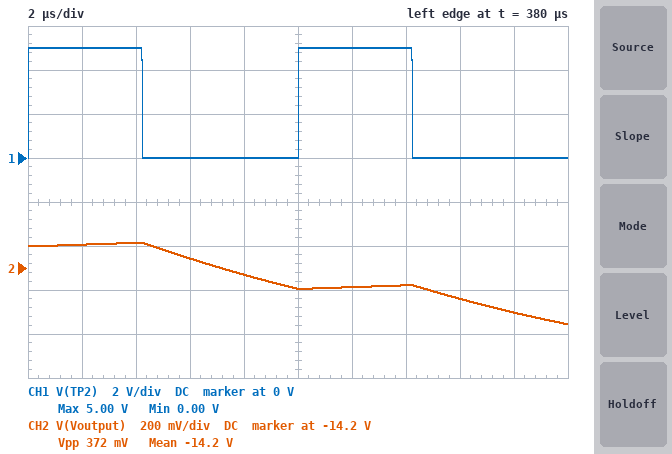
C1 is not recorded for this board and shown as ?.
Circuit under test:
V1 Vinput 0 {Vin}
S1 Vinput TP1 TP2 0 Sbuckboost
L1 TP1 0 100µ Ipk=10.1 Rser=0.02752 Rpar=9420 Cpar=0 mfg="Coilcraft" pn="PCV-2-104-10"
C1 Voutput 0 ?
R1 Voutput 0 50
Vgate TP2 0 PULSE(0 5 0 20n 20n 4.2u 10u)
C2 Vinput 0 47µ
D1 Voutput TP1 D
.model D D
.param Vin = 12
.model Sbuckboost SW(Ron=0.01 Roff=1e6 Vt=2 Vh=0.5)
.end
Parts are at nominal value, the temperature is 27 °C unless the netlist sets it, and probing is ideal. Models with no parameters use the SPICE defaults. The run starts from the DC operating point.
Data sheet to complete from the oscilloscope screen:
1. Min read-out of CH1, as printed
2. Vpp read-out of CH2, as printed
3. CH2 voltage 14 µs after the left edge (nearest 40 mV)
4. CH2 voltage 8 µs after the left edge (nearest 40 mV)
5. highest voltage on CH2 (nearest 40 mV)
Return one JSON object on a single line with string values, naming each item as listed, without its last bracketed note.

{"Min read-out of CH1, as printed": "0.00 V", "Vpp read-out of CH2, as printed": "372 mV", "CH2 voltage 14 µs after the left edge": "-14.28 V", "CH2 voltage 8 µs after the left edge": "-14.24 V", "highest voltage on CH2": "-14.08 V"}
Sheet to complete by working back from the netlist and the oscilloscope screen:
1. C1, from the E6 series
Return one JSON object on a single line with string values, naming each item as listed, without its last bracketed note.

{"C1, from the E6 series": "68 µF"}
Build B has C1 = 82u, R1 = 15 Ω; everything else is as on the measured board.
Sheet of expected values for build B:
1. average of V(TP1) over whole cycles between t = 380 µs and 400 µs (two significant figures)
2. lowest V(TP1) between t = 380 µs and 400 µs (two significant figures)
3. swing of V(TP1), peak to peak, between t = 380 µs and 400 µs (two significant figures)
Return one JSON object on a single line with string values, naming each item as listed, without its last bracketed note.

{"average of V(TP1) over whole cycles between t = 380 µs and 400 µs": "-2.7 V", "lowest V(TP1) between t = 380 µs and 400 µs": "-14 V", "swing of V(TP1), peak to peak, between t = 380 µs and 400 µs": "26 V"}
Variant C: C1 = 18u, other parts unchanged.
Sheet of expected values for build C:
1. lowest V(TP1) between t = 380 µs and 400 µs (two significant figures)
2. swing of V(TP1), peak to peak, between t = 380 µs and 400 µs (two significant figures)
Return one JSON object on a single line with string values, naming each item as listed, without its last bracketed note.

{"lowest V(TP1) between t = 380 µs and 400 µs": "-14 V", "swing of V(TP1), peak to peak, between t = 380 µs and 400 µs": "26 V"}
